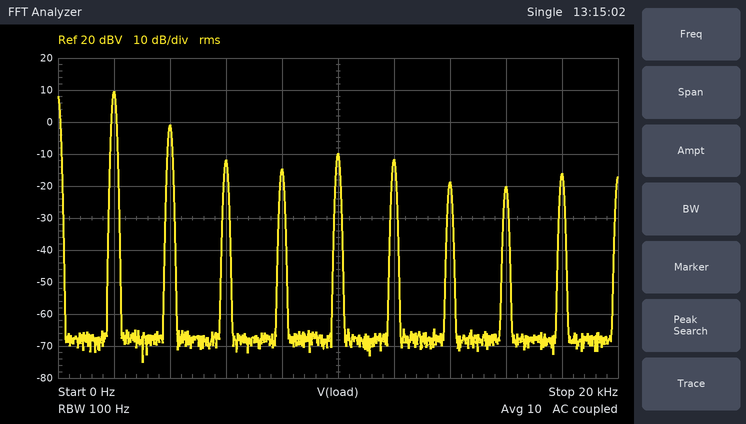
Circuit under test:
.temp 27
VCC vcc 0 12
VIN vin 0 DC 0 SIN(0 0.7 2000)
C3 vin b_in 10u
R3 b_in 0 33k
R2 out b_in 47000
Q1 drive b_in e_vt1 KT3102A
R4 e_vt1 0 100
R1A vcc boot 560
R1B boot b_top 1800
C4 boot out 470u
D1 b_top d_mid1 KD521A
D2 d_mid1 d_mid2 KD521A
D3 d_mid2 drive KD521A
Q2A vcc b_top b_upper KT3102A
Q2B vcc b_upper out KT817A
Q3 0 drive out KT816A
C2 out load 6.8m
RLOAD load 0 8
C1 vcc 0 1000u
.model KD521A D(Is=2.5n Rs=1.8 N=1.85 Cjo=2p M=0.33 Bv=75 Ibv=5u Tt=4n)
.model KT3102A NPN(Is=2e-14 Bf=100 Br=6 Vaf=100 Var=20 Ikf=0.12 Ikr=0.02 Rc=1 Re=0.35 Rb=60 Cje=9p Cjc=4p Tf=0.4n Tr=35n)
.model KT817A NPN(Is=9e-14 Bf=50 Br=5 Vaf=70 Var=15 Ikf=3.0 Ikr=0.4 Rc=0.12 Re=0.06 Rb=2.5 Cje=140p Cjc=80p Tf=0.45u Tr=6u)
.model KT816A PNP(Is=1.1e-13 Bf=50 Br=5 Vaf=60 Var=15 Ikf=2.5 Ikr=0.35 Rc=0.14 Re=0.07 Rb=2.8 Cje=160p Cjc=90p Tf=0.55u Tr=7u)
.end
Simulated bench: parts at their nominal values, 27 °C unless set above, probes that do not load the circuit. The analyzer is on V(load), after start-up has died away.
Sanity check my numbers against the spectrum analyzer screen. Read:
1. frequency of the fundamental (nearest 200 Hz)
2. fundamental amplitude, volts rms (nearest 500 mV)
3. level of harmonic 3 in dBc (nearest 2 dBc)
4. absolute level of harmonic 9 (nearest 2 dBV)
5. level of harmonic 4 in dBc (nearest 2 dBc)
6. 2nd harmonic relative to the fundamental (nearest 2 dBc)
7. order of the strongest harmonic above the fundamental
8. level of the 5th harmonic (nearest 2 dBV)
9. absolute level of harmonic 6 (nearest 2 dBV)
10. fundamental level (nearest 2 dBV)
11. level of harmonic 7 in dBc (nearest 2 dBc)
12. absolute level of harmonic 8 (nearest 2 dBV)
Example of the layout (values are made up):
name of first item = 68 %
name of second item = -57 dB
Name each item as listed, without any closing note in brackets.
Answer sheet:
frequency of the fundamental = 2.0 kHz
fundamental amplitude, volts rms = 3.0 V
level of harmonic 3 in dBc = -22 dBc
absolute level of harmonic 9 = -16 dBV
level of harmonic 4 in dBc = -24 dBc
2nd harmonic relative to the fundamental = -10 dBc
order of the strongest harmonic above the fundamental = 2
level of the 5th harmonic = -10 dBV
absolute level of harmonic 6 = -12 dBV
fundamental level = 10 dBV
level of harmonic 7 in dBc = -28 dBc
absolute level of harmonic 8 = -20 dBV
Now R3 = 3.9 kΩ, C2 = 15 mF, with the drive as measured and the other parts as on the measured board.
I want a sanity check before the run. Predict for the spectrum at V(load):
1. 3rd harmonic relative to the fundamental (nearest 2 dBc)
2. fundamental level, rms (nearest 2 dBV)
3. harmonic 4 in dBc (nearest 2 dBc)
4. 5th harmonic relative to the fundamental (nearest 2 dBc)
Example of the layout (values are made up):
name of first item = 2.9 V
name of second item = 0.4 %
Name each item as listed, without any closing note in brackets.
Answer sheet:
3rd harmonic relative to the fundamental = -18 dBc
fundamental level, rms = 4 dBV
harmonic 4 in dBc = -30 dBc
5th harmonic relative to the fundamental = -26 dBc
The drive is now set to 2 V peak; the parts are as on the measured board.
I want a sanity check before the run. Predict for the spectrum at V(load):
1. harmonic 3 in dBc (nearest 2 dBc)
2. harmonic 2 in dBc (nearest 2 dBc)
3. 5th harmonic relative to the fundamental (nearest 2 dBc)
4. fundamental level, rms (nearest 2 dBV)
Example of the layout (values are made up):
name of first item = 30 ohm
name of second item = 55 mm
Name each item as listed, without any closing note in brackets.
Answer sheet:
harmonic 3 in dBc = -16 dBc
harmonic 2 in dBc = -14 dBc
5th harmonic relative to the fundamental = -24 dBc
fundamental level, rms = 10 dBV
